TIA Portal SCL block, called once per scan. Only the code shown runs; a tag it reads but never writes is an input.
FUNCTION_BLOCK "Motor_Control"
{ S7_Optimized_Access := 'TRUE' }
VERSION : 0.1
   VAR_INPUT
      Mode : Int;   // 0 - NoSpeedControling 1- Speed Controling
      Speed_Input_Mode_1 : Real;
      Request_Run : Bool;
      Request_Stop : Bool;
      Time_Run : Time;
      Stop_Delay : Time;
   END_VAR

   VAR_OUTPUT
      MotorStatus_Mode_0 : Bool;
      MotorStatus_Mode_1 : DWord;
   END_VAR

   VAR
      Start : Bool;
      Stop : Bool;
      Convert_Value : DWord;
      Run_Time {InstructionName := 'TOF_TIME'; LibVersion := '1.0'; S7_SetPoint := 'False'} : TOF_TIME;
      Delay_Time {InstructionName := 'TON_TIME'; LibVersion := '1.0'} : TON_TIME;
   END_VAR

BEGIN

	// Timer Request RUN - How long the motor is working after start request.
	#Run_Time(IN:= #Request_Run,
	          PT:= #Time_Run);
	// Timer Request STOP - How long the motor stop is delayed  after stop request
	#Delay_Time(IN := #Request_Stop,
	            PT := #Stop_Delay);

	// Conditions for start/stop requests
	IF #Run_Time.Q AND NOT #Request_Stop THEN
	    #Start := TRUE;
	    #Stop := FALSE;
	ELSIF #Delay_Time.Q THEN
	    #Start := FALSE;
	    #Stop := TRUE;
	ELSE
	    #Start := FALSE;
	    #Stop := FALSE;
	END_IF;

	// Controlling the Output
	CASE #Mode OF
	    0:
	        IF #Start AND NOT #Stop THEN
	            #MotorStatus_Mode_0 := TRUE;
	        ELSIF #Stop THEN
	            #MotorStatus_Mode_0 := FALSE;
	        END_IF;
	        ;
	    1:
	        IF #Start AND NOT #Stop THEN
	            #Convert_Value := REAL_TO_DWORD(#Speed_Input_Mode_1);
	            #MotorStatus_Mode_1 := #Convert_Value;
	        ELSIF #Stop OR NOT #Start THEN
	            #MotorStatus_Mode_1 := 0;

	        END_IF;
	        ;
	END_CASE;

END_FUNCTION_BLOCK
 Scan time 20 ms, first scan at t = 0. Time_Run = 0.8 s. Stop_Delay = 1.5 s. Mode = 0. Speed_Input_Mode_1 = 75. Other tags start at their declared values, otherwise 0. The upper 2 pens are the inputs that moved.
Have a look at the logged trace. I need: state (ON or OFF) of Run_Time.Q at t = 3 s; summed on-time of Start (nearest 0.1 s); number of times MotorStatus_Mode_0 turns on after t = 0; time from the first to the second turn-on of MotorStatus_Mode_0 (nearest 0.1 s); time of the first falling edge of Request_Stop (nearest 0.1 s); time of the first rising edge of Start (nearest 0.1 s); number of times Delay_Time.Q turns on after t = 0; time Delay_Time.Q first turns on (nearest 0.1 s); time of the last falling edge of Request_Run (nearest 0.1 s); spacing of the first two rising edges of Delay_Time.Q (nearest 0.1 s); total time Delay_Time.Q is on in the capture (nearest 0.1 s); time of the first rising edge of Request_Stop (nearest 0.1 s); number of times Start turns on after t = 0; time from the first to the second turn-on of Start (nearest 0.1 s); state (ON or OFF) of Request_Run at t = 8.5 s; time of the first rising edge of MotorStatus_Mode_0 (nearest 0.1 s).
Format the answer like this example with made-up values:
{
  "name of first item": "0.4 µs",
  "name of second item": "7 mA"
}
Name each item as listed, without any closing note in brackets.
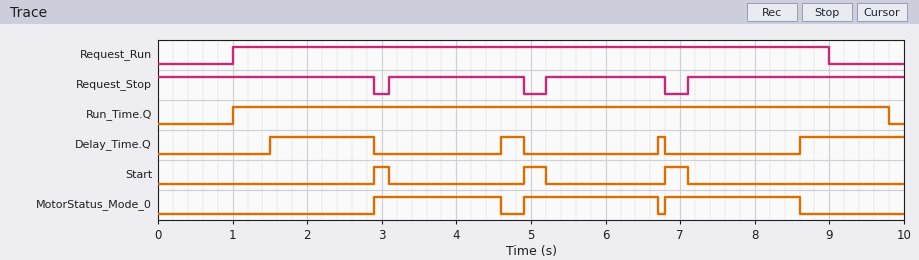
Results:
{
  "state (ON or OFF) of Run_Time.Q at t = 3 s": "ON",
  "summed on-time of Start": "0.8 s",
  "number of times MotorStatus_Mode_0 turns on after t = 0": "3",
  "time from the first to the second turn-on of MotorStatus_Mode_0": "2.0 s",
  "time of the first falling edge of Request_Stop": "2.9 s",
  "time of the first rising edge of Start": "2.9 s",
  "number of times Delay_Time.Q turns on after t = 0": "4",
  "time Delay_Time.Q first turns on": "1.5 s",
  "time of the last falling edge of Request_Run": "9.0 s",
  "spacing of the first two rising edges of Delay_Time.Q": "3.1 s",
  "total time Delay_Time.Q is on in the capture": "3.2 s",
  "time of the first rising edge of Request_Stop": "3.1 s",
  "number of times Start turns on after t = 0": "3",
  "time from the first to the second turn-on of Start": "2.0 s",
  "state (ON or OFF) of Request_Run at t = 8.5 s": "ON",
  "time of the first rising edge of MotorStatus_Mode_0": "2.9 s"
}
